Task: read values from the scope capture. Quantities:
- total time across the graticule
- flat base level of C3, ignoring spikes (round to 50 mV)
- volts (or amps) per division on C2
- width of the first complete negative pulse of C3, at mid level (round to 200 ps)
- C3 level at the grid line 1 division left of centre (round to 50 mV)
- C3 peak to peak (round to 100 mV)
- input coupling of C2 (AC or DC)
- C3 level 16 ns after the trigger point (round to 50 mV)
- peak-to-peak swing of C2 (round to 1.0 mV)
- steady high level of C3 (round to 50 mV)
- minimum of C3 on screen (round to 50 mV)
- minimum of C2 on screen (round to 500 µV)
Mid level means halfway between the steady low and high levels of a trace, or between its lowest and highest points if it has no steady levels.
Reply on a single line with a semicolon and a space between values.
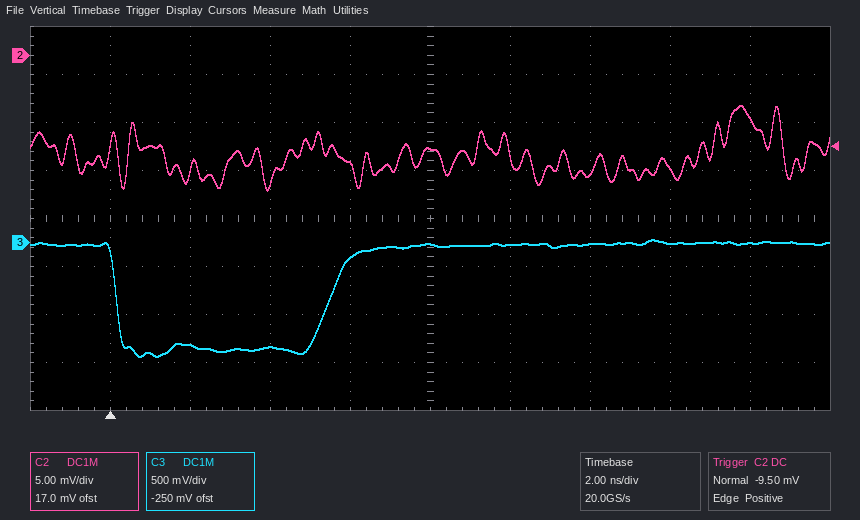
20 ns; -1.10 V; 5 mV; 5.4 ns; -150 mV; 1.20 V; DC; 0 mV; 9.0 mV; 0 mV; -1.20 V; -14.0 mV
